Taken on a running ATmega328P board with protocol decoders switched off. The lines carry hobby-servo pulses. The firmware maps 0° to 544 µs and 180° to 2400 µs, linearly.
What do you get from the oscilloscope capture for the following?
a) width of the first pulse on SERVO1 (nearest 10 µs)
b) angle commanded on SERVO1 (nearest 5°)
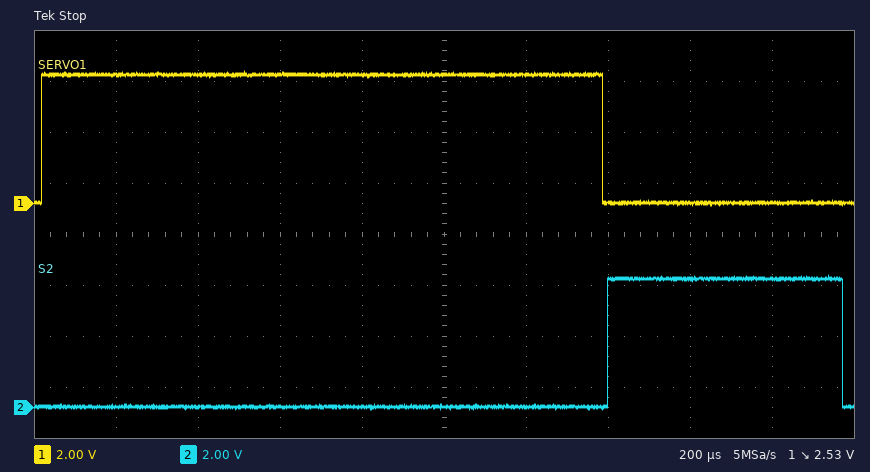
1370 µs
80°
